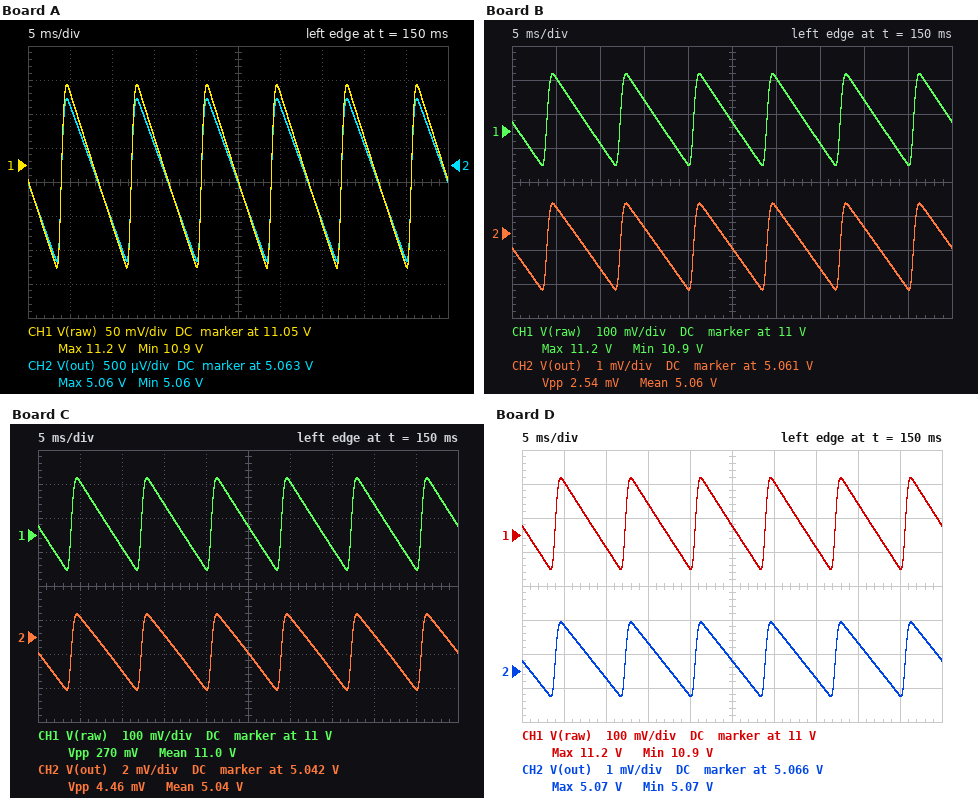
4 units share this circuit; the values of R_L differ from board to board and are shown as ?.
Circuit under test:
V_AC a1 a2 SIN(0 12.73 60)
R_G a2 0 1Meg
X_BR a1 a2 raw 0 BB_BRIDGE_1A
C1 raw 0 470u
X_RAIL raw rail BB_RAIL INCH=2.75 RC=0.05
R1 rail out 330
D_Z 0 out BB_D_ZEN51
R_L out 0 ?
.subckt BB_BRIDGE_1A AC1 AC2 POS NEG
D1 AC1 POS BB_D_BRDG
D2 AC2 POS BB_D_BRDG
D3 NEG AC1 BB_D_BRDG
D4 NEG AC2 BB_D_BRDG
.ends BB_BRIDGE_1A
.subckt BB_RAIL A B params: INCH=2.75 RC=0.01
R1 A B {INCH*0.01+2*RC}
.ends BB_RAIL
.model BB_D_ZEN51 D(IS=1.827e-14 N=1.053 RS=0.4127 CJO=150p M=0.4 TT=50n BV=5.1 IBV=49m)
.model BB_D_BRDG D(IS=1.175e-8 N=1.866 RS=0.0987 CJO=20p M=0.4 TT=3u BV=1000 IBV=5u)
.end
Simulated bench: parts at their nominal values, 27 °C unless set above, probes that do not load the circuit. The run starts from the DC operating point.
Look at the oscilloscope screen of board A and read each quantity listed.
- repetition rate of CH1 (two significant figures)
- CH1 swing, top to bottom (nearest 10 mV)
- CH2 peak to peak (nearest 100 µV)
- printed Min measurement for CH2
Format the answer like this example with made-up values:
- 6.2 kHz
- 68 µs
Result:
- 120 Hz
- 270 mV
- 2.4 mV
- 5.06 V
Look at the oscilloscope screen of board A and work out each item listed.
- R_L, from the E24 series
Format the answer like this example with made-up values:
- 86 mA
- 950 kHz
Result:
- 680 Ω
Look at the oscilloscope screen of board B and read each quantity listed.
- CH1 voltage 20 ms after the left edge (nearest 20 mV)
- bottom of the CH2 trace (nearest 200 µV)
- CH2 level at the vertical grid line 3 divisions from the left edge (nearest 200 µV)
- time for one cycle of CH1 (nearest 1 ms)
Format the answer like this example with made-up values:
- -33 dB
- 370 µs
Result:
- 10.90 V
- 5.0594 V
- 5.0612 V
- 8 ms
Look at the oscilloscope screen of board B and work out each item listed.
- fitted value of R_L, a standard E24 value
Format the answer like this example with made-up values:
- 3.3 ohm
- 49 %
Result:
- 620 Ω
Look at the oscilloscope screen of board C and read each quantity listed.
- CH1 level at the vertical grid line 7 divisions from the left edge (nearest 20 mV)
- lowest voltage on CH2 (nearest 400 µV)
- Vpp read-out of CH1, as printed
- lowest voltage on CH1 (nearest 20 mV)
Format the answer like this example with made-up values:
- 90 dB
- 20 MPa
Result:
- 10.96 V
- 5.0388 V
- 270 mV
- 10.90 V
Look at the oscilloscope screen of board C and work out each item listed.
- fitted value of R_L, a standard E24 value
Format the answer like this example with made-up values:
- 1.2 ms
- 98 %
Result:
- 390 Ω
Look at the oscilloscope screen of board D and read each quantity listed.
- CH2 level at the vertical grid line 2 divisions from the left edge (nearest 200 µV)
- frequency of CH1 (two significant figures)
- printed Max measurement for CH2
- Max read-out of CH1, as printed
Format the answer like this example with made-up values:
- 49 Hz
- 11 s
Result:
- 5.0658 V
- 120 Hz
- 5.07 V
- 11.2 V
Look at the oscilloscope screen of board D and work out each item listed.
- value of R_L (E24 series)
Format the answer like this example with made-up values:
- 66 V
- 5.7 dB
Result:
- 820 Ω
